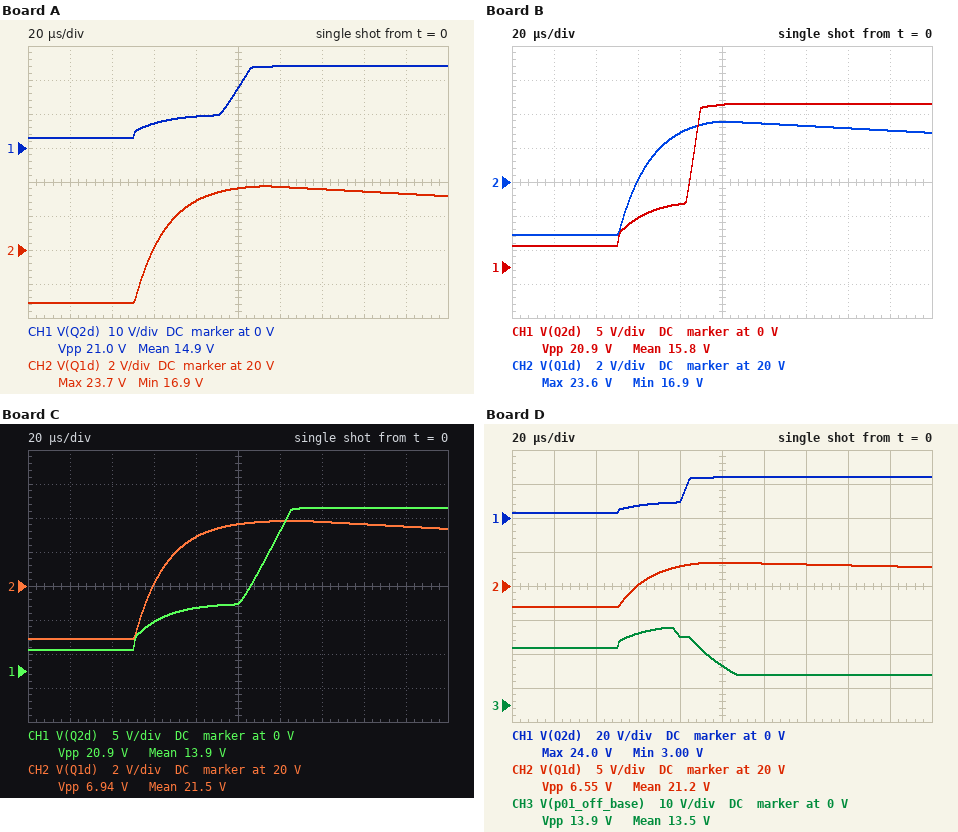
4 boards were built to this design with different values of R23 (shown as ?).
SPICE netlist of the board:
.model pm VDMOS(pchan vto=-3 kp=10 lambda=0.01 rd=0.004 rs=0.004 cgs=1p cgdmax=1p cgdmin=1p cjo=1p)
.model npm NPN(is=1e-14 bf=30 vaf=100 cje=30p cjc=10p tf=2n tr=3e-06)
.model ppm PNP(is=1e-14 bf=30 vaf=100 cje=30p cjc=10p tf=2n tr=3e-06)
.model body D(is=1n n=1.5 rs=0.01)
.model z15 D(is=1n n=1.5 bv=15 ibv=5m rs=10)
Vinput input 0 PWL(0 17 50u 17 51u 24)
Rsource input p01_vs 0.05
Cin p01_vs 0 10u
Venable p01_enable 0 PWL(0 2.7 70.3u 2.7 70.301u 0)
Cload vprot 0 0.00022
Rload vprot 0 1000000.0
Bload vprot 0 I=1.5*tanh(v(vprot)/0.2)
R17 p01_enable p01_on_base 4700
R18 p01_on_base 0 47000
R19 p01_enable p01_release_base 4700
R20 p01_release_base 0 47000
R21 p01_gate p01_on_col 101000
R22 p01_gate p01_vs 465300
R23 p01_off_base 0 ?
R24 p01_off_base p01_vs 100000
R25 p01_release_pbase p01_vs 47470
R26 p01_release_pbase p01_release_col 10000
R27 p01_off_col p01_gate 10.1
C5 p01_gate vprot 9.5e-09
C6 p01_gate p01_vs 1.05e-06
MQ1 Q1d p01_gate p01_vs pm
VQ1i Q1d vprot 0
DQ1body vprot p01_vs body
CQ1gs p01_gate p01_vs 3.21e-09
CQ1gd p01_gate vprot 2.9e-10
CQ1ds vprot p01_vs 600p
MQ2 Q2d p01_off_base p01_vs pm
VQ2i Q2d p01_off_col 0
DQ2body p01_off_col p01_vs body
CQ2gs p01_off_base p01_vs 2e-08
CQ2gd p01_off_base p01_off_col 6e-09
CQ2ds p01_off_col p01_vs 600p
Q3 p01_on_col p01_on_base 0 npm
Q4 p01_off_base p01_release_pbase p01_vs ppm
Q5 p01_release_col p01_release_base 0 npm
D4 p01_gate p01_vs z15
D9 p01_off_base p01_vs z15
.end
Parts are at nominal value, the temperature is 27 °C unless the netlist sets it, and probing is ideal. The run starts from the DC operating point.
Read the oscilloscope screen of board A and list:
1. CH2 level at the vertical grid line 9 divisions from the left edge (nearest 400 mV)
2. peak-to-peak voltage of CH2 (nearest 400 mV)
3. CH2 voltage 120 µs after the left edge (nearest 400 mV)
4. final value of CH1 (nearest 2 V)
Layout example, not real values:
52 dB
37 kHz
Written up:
23.2 V
6.8 V
23.6 V
24 V
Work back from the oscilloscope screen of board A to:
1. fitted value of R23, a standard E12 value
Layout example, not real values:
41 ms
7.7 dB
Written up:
3.3 kΩ
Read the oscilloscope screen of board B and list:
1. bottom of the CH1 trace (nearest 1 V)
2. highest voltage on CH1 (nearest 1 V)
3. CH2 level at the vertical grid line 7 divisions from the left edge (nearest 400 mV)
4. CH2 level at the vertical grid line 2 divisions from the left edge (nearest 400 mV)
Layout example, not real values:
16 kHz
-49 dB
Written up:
3 V
24 V
23.2 V
16.8 V
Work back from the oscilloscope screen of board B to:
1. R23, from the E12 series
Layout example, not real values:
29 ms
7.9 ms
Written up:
1.5 kΩ
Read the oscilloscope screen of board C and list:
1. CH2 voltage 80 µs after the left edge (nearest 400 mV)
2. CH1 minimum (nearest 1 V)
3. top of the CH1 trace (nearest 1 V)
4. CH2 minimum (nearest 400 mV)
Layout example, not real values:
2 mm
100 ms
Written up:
22.8 V
3 V
24 V
16.8 V
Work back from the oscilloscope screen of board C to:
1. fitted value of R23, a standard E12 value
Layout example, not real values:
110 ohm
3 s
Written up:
5.6 kΩ
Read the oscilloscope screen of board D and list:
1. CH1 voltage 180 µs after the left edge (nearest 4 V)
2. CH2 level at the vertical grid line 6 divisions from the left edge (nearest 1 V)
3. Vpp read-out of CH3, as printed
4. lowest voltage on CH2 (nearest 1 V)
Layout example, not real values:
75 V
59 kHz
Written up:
24 V
23 V
13.9 V
17 V
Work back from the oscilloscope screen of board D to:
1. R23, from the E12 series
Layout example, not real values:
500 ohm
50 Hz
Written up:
1 kΩ
